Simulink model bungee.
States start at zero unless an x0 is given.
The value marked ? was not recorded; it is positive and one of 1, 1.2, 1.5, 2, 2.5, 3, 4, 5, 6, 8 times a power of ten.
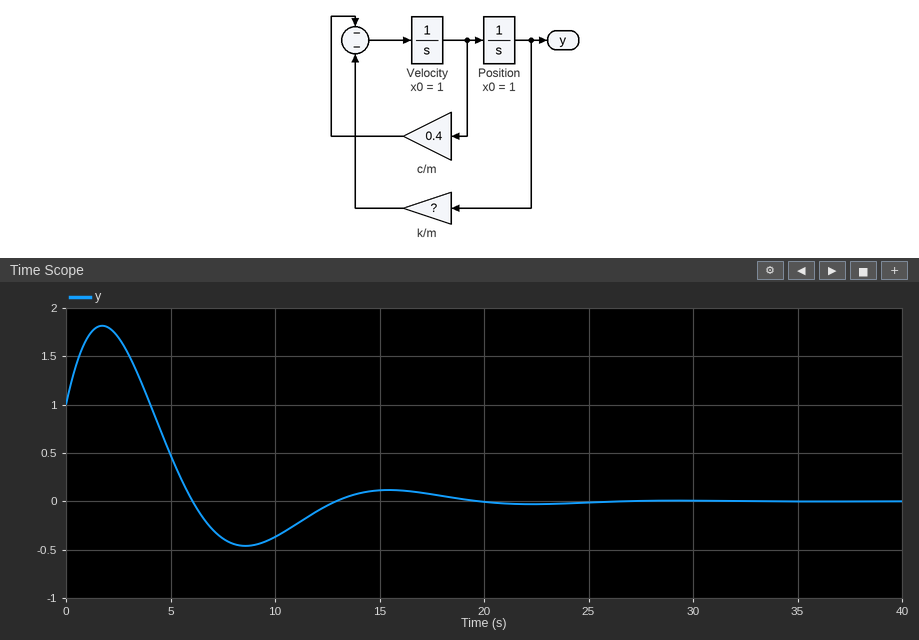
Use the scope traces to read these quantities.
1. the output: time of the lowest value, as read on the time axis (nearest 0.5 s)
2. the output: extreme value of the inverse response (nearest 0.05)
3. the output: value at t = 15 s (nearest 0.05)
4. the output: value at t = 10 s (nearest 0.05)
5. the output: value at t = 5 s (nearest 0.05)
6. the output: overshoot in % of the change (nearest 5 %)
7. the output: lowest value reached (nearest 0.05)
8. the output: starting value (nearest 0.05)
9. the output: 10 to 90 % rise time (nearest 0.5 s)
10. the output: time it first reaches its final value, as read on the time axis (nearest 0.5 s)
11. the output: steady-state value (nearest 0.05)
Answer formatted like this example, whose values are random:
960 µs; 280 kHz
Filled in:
8.5 s; 1.80; 0.10; -0.35; 0.50; 45 %; -0.45; 1.00; 1.5 s; 6.0 s; 0.00
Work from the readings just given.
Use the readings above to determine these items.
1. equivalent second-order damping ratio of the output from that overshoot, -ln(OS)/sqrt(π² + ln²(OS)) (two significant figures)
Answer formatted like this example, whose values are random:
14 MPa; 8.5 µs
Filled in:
0.25
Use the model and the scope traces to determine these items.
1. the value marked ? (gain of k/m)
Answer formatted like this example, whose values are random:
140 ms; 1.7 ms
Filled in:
0.25
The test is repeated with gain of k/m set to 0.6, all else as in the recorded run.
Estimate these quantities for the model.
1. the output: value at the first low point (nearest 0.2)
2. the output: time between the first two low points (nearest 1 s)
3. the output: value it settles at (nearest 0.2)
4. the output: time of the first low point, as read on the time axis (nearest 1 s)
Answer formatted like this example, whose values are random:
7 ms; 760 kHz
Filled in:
-0.6; 8 s; 0.0; 5 s
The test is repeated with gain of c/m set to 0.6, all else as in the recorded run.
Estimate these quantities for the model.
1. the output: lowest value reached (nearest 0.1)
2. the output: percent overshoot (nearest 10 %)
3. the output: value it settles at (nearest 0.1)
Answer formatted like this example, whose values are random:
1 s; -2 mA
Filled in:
-0.2; 20 %; 0.0
